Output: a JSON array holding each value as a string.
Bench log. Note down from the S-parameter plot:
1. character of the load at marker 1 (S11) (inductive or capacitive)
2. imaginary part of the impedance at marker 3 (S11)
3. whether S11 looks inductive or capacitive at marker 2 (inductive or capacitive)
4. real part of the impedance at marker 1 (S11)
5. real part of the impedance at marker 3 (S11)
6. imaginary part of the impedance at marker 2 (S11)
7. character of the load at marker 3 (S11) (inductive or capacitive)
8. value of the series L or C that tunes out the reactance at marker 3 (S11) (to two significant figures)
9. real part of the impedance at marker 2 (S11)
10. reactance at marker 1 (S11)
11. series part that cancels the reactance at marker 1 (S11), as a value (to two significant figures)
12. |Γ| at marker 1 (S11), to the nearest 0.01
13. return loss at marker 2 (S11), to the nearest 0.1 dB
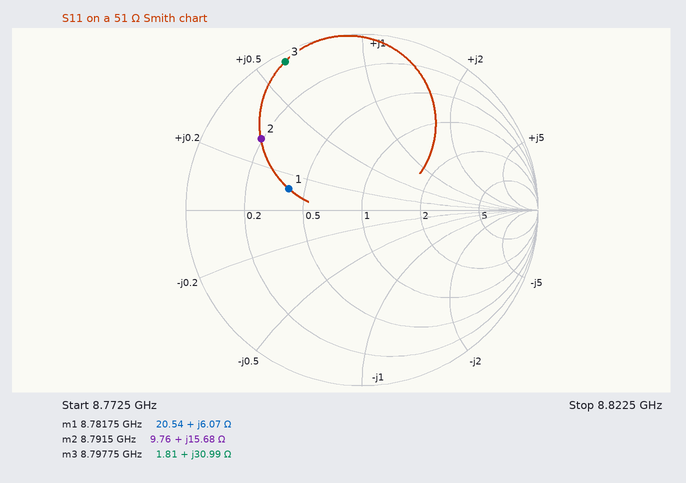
["inductive", "+30.99 Ω", "inductive", "20.54 Ω", "1.81 Ω", "+15.68 Ω", "inductive", "580 fF", "9.76 Ω", "+6.07 Ω", "3.0 pF", "0.43", "3.1 dB"]
